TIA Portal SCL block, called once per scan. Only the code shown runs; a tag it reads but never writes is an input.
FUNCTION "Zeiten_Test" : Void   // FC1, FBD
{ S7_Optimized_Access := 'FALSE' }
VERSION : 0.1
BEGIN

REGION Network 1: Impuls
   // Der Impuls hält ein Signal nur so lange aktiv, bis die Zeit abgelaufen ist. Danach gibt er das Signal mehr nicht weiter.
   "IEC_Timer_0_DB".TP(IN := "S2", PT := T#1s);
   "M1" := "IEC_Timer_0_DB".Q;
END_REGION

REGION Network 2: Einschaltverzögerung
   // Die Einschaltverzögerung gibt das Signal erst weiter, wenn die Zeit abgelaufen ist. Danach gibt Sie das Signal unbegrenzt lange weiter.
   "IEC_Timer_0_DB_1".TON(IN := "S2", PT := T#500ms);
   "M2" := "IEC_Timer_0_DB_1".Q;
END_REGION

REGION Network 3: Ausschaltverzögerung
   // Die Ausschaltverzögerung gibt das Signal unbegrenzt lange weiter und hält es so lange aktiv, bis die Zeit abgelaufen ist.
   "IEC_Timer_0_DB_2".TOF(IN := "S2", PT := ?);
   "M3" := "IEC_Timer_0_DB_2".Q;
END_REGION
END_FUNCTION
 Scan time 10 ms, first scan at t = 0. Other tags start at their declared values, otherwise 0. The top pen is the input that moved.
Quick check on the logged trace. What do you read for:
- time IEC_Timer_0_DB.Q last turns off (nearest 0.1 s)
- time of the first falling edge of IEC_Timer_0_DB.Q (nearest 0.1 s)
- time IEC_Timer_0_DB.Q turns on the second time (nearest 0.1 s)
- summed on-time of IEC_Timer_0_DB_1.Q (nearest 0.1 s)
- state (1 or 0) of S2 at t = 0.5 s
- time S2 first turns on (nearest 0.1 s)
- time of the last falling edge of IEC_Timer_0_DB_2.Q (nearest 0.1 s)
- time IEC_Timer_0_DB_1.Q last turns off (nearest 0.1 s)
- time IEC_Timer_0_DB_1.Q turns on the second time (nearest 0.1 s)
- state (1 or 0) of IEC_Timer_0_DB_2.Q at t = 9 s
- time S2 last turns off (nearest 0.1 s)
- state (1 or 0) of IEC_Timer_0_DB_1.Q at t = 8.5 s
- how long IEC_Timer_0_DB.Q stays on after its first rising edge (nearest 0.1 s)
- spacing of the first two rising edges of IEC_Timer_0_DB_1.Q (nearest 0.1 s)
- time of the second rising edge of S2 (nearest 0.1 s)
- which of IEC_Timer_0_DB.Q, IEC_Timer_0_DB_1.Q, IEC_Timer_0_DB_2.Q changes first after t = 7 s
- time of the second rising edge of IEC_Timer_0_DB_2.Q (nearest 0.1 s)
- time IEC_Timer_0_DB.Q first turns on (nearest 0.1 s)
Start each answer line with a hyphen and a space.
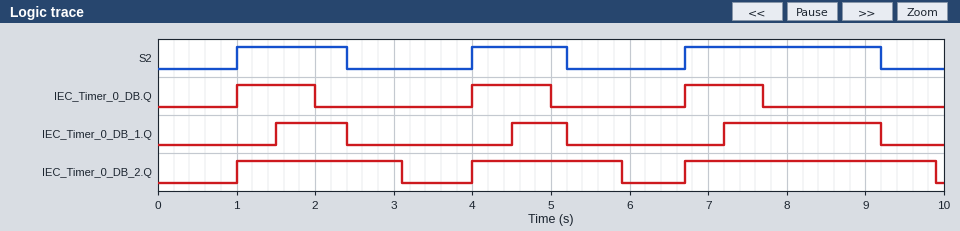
- 7.7 s
- 2.0 s
- 4.0 s
- 3.6 s
- 0
- 1.0 s
- 9.9 s
- 9.2 s
- 4.5 s
- 1
- 9.2 s
- 1
- 1.0 s
- 3.0 s
- 4.0 s
- IEC_Timer_0_DB_1.Q
- 4.0 s
- 1.0 s
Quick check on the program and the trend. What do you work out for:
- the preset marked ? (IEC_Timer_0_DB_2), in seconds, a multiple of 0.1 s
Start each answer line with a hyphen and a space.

- 0.7 s
